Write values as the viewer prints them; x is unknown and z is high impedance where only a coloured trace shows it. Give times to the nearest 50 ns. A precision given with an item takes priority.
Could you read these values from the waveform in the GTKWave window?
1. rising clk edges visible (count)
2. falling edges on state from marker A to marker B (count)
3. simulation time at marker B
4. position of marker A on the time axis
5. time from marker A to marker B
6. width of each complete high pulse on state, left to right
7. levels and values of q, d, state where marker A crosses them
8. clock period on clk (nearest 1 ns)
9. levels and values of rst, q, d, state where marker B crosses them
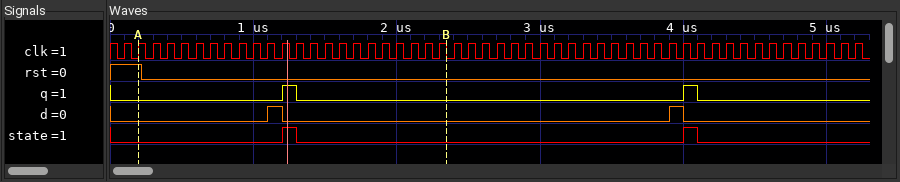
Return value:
52
1
2350 ns
200 ns
2150 ns
100 ns, 100 ns
q=0, d=0, state=0
100 ns
rst=0, q=0, d=0, state=0
